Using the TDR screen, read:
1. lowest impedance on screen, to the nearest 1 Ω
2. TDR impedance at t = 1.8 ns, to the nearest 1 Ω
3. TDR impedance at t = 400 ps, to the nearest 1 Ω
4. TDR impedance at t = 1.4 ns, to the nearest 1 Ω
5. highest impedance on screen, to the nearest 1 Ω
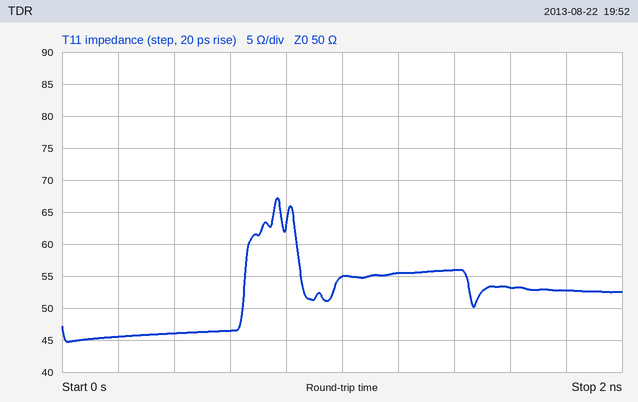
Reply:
45 Ω
53 Ω
46 Ω
56 Ω
67 Ω
